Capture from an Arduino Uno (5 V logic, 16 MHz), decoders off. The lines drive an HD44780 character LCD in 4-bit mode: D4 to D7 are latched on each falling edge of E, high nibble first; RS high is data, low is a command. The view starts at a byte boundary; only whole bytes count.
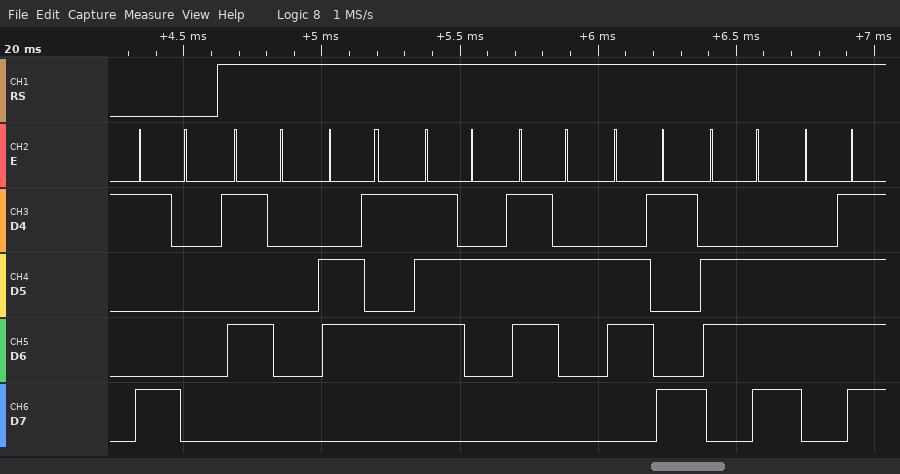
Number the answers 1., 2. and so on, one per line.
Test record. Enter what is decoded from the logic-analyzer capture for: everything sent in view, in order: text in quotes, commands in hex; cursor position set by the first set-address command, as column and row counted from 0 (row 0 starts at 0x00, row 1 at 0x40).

1. 0x90 "Perrino"
2. column 16, row 0
